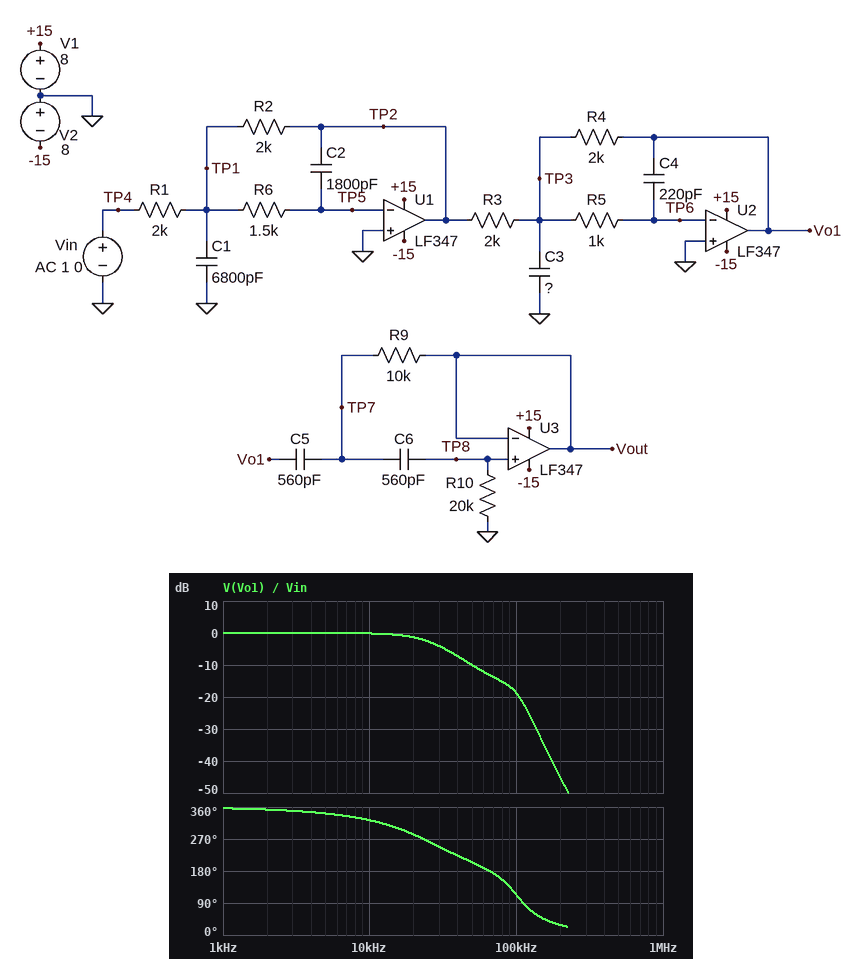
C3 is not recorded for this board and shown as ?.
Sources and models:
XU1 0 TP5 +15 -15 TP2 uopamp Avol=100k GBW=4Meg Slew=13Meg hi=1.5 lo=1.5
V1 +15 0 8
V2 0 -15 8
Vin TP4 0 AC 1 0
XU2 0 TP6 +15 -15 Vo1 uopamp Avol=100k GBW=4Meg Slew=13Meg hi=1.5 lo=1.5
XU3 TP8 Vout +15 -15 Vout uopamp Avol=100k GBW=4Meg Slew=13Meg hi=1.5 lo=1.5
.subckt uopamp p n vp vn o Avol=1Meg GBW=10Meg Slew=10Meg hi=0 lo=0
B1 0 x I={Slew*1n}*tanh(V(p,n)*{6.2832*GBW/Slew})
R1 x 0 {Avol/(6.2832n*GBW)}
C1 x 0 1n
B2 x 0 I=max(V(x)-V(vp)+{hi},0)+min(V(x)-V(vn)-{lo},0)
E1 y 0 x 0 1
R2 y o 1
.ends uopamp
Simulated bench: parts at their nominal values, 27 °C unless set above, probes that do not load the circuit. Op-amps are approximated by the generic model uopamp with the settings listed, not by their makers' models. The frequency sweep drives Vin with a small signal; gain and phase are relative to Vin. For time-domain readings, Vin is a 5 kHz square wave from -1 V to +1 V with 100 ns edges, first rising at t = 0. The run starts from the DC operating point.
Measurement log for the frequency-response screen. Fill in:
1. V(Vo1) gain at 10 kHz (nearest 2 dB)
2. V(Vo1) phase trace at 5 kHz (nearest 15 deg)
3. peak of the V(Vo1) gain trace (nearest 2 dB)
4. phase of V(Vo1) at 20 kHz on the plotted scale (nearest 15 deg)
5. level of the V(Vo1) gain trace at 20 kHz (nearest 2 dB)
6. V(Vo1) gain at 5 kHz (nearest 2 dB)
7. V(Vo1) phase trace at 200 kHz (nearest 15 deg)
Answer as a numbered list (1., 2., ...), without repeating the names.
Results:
1. 0 dB
2. 345 deg
3. 0 dB
4. 285 deg
5. -2 dB
6. 0 dB
7. 30 deg
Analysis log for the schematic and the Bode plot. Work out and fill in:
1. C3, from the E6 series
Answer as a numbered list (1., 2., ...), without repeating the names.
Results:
1. 4.7 nF
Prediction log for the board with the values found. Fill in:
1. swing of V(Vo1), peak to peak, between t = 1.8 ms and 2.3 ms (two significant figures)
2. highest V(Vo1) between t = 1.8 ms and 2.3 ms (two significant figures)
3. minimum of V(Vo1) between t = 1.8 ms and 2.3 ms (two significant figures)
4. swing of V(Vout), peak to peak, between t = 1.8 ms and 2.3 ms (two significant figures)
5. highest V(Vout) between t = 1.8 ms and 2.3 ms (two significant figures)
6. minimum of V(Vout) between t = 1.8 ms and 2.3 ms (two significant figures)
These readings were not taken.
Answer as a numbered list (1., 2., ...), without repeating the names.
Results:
1. 2.1 V
2. 1.1 V
3. -1.1 V
4. 1.1 V
5. 560 mV
6. -560 mV
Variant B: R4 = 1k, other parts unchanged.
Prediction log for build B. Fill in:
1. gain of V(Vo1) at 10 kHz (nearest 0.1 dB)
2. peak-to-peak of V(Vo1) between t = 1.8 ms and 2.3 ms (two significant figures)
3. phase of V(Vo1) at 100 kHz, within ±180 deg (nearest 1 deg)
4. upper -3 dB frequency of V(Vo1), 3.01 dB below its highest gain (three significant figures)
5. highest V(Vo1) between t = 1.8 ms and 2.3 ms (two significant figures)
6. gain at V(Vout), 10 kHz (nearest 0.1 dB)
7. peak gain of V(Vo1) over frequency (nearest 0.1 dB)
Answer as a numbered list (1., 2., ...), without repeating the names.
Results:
1. -6.2 dB
2. 1.1 V
3. 165 deg
4. 25.6 kHz
5. 530 mV
6. -18.6 dB
7. -6.0 dB
